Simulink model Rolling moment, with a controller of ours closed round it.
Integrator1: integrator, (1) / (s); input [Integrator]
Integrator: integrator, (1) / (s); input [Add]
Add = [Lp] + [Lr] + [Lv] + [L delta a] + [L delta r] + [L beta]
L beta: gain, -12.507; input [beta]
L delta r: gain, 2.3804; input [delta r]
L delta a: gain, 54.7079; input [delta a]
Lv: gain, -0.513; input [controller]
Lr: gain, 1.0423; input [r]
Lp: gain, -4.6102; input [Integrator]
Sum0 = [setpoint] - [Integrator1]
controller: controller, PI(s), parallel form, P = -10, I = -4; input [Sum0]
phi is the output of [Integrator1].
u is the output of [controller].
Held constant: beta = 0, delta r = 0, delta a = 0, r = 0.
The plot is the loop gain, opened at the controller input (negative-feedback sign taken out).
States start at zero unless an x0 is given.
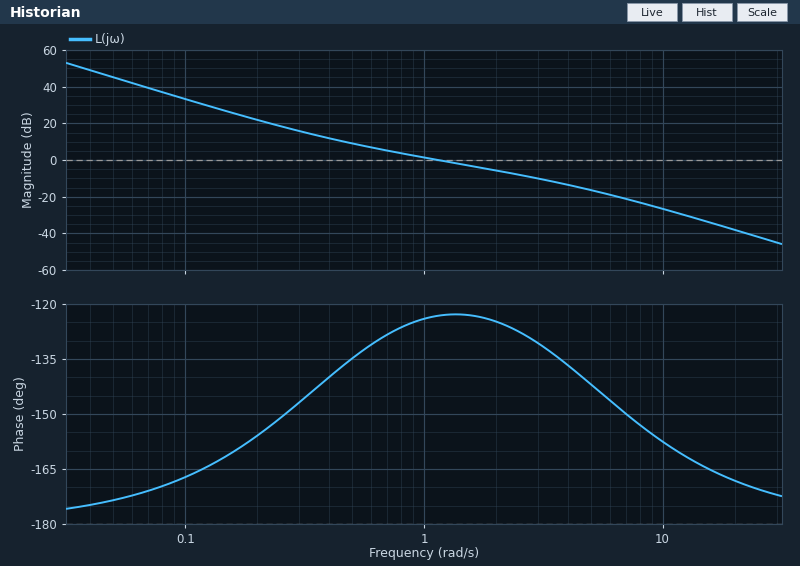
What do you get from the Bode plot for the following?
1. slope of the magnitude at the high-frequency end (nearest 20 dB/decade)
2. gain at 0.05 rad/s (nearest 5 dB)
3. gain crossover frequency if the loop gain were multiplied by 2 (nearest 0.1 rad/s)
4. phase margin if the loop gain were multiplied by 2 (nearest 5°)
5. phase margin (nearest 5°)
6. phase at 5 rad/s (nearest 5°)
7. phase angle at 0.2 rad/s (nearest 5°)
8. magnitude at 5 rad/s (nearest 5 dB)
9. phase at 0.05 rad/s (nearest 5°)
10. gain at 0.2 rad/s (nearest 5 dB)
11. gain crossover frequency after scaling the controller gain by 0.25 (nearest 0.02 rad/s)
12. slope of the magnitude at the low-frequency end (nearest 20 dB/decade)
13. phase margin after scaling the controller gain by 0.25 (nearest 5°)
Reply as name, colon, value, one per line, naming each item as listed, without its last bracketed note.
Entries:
slope of the magnitude at the high-frequency end: -40 dB/decade
gain at 0.05 rad/s: 45 dB
gain crossover frequency if the loop gain were multiplied by 2: 2.1 rad/s
phase margin if the loop gain were multiplied by 2: 55°
phase margin: 55°
phase at 5 rad/s: -140°
phase angle at 0.2 rad/s: -155°
magnitude at 5 rad/s: -15 dB
phase at 0.05 rad/s: -175°
gain at 0.2 rad/s: 20 dB
gain crossover frequency after scaling the controller gain by 0.25: 0.40 rad/s
slope of the magnitude at the low-frequency end: -40 dB/decade
phase margin after scaling the controller gain by 0.25: 40°
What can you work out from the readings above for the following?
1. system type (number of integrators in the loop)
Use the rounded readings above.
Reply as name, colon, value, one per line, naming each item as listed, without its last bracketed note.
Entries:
system type: 2
